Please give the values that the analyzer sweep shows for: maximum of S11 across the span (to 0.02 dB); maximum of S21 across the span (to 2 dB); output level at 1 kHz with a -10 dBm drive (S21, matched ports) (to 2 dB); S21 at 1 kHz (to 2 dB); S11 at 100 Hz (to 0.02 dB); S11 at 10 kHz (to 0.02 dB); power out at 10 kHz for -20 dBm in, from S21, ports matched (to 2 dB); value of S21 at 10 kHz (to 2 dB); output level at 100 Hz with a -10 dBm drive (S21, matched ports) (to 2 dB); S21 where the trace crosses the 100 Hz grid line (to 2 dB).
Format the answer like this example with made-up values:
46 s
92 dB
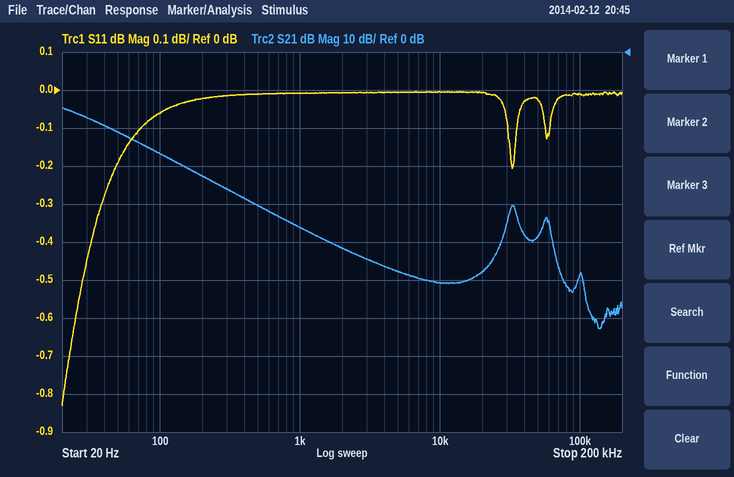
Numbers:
0.00 dB
-14 dB
-56 dBm
-46 dB
-0.06 dB
0.00 dB
-80 dBm
-60 dB
-36 dBm
-26 dB
